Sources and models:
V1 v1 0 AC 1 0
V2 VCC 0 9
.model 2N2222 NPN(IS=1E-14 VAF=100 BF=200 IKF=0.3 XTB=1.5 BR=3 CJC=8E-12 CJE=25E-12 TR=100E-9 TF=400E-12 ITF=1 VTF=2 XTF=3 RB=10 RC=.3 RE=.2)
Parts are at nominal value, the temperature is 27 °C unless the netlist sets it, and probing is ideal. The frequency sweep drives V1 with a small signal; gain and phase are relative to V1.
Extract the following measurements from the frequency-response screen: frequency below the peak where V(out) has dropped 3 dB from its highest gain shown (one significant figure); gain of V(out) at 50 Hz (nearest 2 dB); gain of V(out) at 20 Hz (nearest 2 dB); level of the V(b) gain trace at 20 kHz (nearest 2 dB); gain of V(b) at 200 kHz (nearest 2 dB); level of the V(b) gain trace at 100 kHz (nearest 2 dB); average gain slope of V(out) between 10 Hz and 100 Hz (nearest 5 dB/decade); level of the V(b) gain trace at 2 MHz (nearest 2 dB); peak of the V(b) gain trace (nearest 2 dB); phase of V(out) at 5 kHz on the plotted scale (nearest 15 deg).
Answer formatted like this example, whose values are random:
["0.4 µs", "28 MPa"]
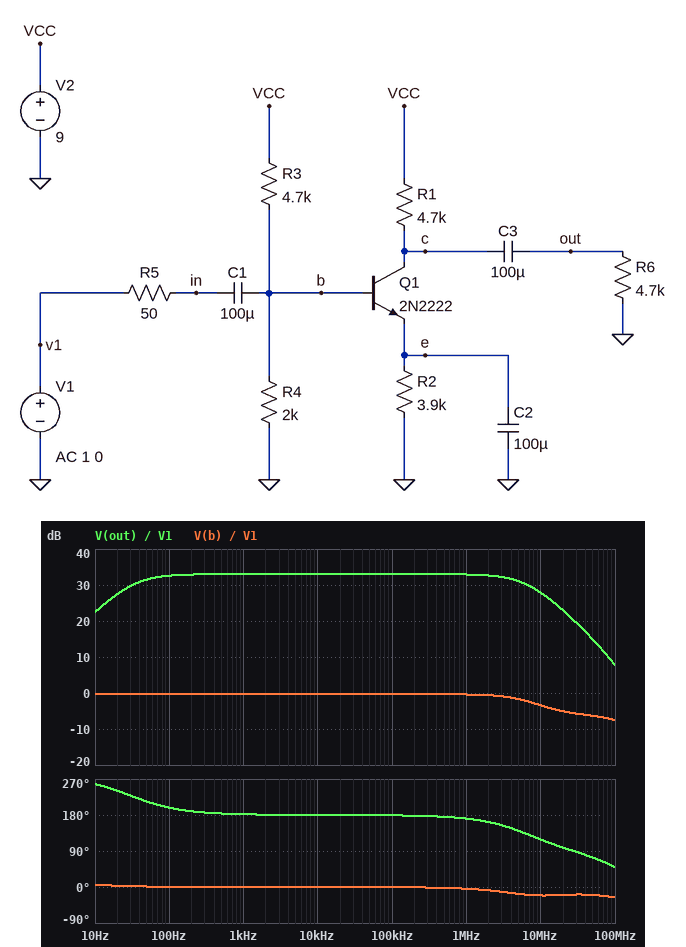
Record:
["30 Hz", "32 dB", "28 dB", "0 dB", "0 dB", "0 dB", "10 dB/decade", "0 dB", "0 dB", "180 deg"]
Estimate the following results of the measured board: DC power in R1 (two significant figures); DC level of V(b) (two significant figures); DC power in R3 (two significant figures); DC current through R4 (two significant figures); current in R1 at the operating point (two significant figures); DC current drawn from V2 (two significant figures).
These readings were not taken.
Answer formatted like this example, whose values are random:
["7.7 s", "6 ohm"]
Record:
["1.3 mW", "2.7 V", "8.5 mW", "1.3 mA", "520 µA", "1.9 mA"]
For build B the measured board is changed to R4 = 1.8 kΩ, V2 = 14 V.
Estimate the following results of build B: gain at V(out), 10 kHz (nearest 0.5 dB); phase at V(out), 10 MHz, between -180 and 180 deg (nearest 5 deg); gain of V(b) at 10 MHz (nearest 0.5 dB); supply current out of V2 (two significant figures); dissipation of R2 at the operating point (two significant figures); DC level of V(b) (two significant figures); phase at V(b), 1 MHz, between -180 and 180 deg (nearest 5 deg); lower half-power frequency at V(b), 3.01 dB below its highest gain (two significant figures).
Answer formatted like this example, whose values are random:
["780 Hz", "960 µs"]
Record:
["37.0 dB", "115 deg", "-4.5 dB", "3.0 mA", "2.7 mW", "3.9 V", "-5 deg", "1.2 Hz"]
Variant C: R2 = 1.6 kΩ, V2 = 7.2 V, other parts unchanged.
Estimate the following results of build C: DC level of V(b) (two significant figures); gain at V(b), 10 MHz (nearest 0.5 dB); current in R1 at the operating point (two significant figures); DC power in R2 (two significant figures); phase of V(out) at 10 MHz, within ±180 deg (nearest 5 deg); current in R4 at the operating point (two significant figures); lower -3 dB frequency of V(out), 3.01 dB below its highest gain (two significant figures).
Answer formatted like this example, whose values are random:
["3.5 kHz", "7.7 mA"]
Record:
["2.1 V", "-6.0 dB", "930 µA", "1.4 mW", "105 deg", "1.1 mA", "56 Hz"]
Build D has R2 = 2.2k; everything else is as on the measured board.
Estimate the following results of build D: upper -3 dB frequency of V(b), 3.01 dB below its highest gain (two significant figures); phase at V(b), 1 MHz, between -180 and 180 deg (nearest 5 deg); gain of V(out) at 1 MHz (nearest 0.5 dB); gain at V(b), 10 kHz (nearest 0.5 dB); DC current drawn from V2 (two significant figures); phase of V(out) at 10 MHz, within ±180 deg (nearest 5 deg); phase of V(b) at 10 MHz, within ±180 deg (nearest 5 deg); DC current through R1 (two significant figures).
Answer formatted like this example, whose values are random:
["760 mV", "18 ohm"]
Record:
["5.1 MHz", "-10 deg", "37.5 dB", "-0.5 dB", "2.3 mA", "110 deg", "-25 deg", "920 µA"]
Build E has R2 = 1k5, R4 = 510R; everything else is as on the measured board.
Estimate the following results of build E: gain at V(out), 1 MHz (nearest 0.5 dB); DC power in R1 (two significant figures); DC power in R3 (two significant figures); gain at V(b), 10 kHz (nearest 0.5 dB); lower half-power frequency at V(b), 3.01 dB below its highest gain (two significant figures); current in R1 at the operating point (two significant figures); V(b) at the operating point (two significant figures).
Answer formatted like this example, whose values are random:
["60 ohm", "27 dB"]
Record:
["23.5 dB", "150 µW", "14 mW", "-1.0 dB", "3.1 Hz", "180 µA", "880 mV"]
